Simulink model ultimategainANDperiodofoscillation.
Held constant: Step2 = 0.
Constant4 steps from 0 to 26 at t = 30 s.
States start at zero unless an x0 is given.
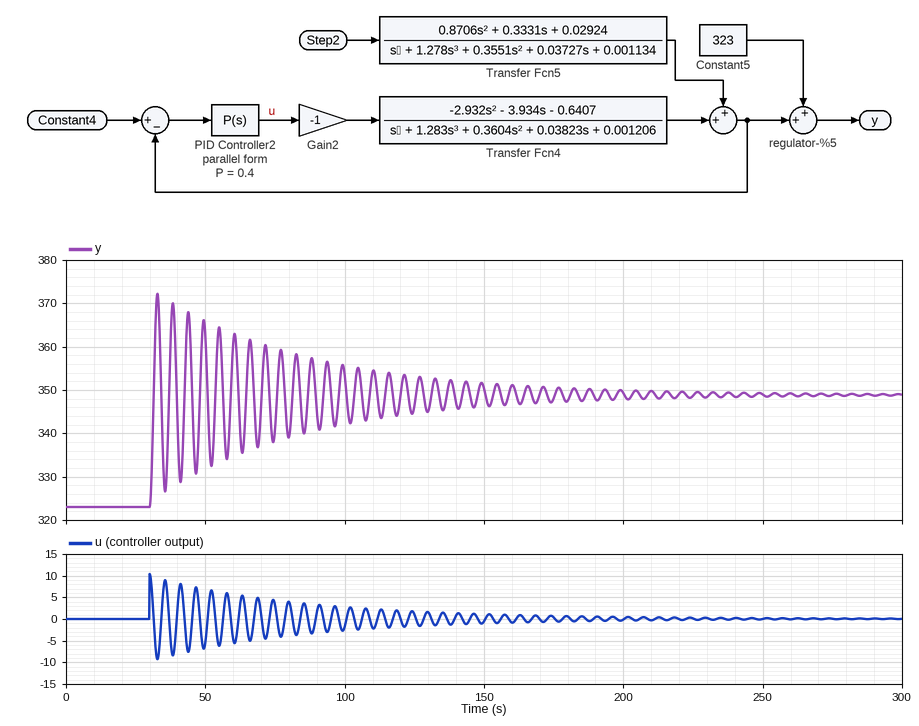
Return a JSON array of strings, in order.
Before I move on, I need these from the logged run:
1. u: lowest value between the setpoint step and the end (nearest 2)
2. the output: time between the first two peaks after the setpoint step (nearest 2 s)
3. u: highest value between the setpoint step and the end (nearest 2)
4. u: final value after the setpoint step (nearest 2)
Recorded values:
["-10", "6 s", "10", "0"]
